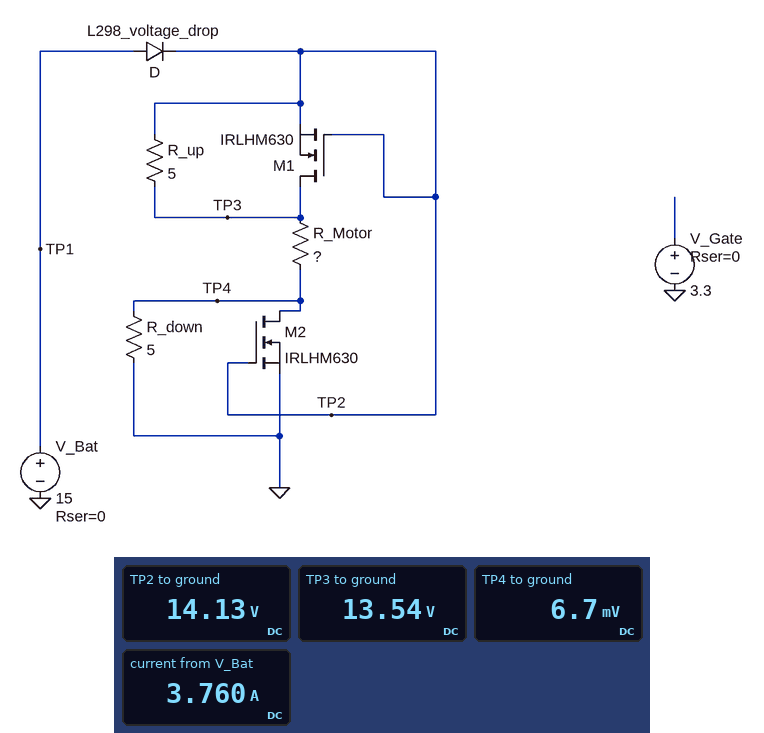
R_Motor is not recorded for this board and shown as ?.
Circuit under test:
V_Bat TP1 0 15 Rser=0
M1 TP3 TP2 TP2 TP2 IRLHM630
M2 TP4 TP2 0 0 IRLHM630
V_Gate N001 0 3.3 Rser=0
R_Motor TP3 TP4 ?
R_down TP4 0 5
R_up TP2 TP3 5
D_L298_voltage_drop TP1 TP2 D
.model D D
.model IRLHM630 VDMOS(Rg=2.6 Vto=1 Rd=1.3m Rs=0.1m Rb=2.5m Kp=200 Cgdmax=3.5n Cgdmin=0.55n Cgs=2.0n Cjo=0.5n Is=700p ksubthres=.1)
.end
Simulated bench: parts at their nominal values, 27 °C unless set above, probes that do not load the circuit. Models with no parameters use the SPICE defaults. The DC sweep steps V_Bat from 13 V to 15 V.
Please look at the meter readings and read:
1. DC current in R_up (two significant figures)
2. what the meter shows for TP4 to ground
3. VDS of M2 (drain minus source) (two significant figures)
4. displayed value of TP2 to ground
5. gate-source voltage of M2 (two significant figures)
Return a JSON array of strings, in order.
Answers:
["120 mA", "6.7 mV", "6.7 mV", "14.13 V", "14 V"]
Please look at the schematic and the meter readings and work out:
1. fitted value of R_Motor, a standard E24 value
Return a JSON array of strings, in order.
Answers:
["3.6 Ω"]
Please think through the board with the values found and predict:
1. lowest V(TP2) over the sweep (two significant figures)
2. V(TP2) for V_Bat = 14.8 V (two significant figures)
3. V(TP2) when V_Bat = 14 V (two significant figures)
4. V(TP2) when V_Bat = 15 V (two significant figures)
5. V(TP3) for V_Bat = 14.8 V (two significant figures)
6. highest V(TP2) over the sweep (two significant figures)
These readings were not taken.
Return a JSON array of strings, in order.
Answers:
["12 V", "14 V", "13 V", "14 V", "13 V", "14 V"]
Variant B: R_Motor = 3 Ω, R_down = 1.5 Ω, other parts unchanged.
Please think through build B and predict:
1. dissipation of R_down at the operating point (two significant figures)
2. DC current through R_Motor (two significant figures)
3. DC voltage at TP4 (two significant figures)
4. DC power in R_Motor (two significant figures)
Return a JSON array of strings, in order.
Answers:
["43 µW", "4.5 A", "8.0 mV", "61 W"]
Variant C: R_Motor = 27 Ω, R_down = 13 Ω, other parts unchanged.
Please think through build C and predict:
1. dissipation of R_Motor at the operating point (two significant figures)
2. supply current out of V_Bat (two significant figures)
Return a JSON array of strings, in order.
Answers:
["6.9 W", "510 mA"]
